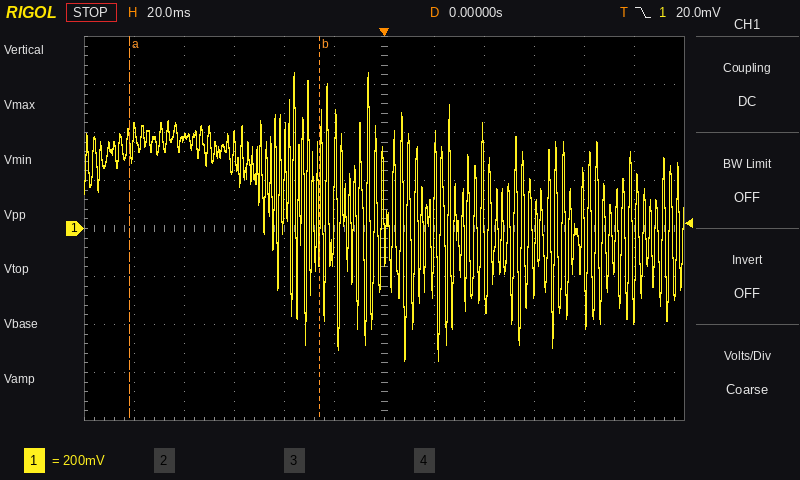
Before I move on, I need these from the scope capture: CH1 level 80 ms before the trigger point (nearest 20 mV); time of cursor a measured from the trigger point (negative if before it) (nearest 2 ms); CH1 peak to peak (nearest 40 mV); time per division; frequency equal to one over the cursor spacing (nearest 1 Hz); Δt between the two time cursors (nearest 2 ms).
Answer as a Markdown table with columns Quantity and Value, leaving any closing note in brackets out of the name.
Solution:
| Quantity | Value |
|---|---|
| CH1 level 80 ms before the trigger point | 380 mV |
| time of cursor a measured from the trigger point (negative if before it) | -102 ms |
| CH1 peak to peak | 1.20 V |
| time per division | 20 ms |
| frequency equal to one over the cursor spacing | 13 Hz |
| Δt between the two time cursors | 76 ms |
